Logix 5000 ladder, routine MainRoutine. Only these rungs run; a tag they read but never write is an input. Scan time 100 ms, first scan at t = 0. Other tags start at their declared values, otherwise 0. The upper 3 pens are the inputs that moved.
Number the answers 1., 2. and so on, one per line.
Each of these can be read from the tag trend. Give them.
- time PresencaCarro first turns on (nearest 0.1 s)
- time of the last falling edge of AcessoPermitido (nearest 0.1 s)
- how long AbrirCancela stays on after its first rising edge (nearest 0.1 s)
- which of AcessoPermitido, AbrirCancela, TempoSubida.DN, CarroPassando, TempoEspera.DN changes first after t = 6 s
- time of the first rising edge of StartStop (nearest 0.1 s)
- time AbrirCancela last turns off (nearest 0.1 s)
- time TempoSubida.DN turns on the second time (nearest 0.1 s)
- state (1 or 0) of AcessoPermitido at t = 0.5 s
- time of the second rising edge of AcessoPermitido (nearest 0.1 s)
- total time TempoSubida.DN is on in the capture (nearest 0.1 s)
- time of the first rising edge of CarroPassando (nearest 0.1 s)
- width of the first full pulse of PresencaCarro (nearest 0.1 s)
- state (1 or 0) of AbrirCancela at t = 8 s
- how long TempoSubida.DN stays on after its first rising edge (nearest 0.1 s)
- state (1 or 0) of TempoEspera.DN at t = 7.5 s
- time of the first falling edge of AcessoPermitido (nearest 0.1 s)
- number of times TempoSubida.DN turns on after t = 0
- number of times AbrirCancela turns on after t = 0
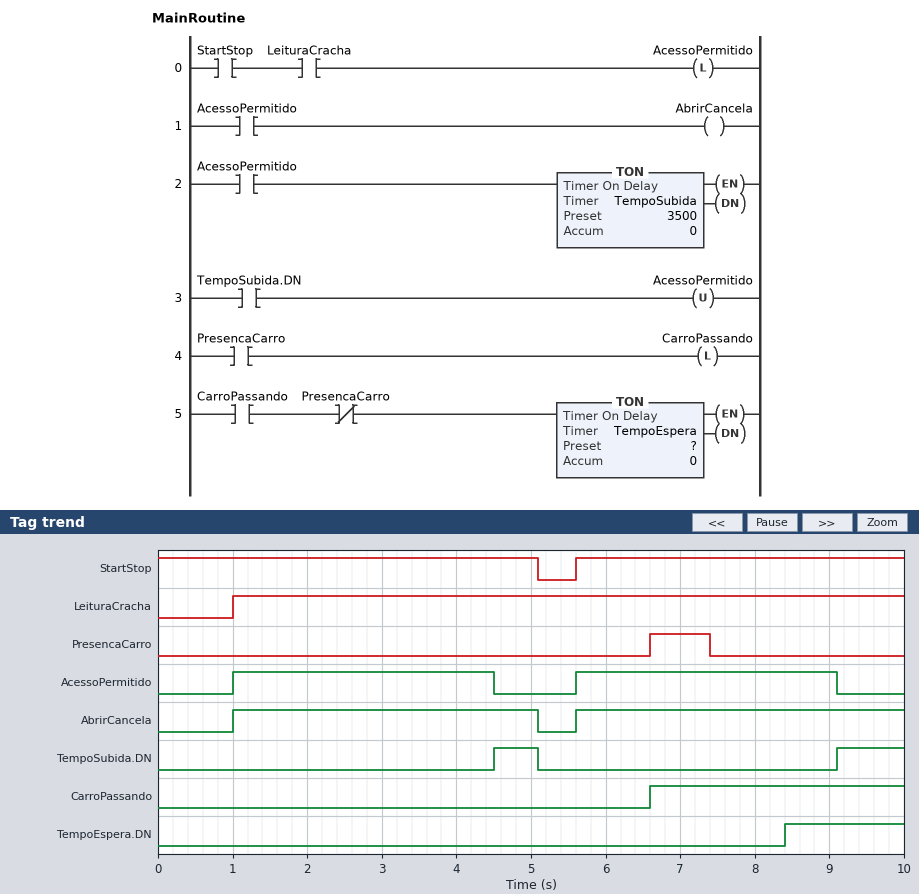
1. 6.6 s
2. 9.1 s
3. 4.1 s
4. CarroPassando
5. 5.6 s
6. 5.1 s
7. 9.1 s
8. 0
9. 5.6 s
10. 1.5 s
11. 6.6 s
12. 0.8 s
13. 1
14. 0.6 s
15. 0
16. 4.5 s
17. 2
18. 2
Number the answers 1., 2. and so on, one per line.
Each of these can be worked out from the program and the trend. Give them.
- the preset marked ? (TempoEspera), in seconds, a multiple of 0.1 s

1. 1.0 s
